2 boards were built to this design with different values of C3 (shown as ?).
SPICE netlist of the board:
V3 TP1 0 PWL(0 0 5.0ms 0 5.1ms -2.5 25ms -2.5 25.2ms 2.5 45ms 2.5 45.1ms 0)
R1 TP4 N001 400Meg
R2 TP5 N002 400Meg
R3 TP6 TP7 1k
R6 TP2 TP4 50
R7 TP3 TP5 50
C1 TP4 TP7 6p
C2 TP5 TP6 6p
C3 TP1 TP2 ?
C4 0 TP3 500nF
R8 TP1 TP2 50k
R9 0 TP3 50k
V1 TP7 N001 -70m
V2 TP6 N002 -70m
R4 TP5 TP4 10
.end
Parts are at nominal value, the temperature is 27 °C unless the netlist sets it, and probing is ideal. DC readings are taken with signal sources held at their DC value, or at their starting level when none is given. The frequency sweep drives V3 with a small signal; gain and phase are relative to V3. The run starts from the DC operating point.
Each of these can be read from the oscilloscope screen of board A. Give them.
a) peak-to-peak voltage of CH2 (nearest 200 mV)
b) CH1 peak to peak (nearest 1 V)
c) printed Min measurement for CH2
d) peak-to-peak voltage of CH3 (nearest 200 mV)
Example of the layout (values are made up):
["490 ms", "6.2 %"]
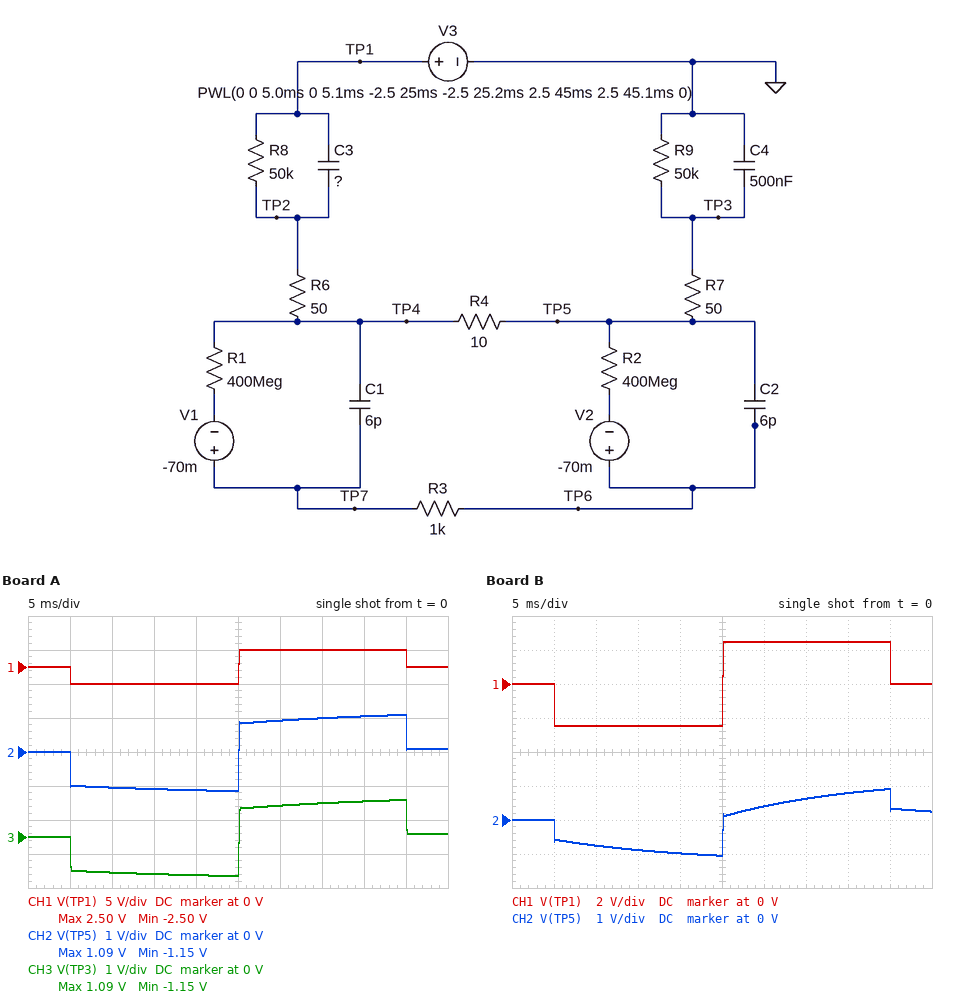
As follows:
["2.2 V", "5 V", "-1.15 V", "2.2 V"]
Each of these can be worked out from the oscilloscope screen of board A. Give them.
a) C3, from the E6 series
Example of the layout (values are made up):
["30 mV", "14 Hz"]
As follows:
["330 nF"]
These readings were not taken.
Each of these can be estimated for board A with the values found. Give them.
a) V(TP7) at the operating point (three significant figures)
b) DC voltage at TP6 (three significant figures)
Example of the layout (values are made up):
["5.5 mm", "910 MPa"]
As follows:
["-70.0 mV", "-70.0 mV"]
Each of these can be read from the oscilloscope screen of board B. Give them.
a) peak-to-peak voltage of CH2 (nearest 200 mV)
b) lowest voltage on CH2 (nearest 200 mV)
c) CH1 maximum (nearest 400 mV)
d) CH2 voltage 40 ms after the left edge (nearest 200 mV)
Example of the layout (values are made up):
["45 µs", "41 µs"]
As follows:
["2.0 V", "-1.0 V", "2.4 V", "800 mV"]
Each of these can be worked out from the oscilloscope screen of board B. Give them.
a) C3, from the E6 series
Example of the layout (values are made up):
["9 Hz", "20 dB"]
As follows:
["150 nF"]
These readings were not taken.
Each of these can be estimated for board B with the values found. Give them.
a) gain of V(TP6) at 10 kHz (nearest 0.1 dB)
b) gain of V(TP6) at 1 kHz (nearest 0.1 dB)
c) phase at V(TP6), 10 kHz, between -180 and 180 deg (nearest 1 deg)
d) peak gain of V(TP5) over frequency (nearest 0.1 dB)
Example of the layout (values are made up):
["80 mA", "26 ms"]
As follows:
["-8.9 dB", "-12.6 dB", "21 deg", "-6.0 dB"]
